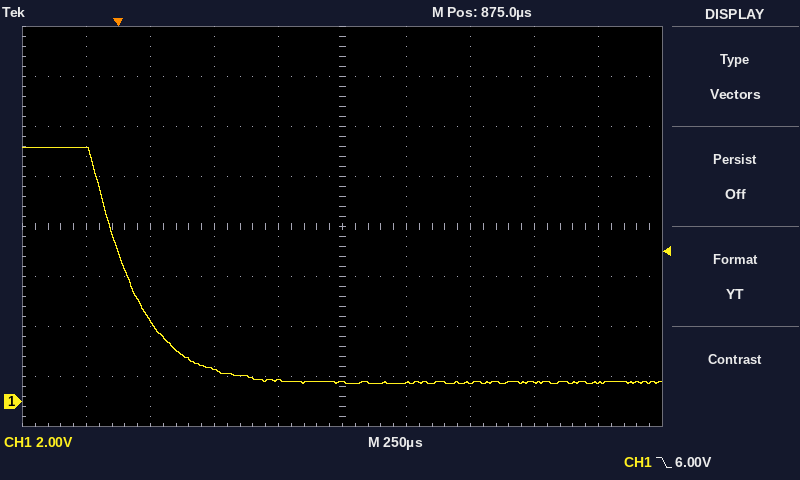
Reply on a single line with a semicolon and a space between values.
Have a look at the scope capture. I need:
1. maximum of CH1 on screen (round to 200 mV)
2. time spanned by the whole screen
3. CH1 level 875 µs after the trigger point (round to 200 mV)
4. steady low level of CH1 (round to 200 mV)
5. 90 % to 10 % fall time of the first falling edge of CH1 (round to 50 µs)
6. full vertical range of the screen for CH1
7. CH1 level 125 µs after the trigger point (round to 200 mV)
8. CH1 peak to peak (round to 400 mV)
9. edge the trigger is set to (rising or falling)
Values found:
10.2 V; 2.5 ms; 800 mV; 800 mV; 350 µs; 16 V; 3.2 V; 9.6 V; falling
